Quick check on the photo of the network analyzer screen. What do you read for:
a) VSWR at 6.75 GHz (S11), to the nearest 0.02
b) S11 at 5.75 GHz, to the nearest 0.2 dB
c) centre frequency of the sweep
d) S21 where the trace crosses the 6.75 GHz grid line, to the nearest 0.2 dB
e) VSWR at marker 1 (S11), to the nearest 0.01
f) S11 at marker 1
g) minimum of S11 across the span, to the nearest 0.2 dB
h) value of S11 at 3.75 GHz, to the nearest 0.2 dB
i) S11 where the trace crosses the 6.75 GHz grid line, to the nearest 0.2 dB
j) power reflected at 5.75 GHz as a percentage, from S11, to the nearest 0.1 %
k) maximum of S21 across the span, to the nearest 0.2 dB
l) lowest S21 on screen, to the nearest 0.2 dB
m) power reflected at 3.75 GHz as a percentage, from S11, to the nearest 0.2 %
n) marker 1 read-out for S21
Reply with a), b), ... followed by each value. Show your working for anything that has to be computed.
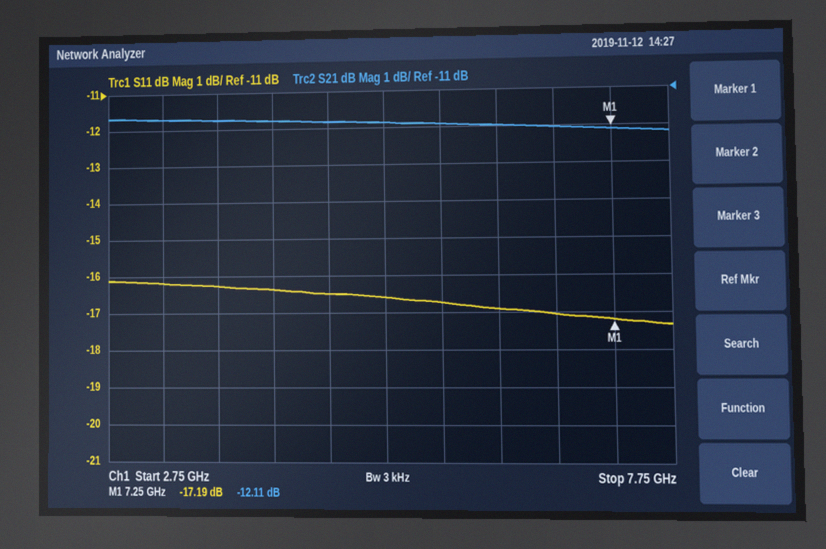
a) |Γ| = 10^(-17/20) = 0.1413; VSWR = (1 + 0.1413)/(1 − 0.1413) ≈ 1.33, so 1.32 to the nearest 0.02
b) -16.8 dB
c) 5.25 GHz
d) -12.0 dB
e) (1 + 0.1382)/(1 − 0.1382) ≈ 1.32
f) -17.19 dB
g) -17.4 dB
h) -16.2 dB
i) -17.0 dB
j) 10^(-16.8/10) ≈ 2.1 %
k) -11.6 dB
l) -12.2 dB
m) 10^(-16.2/10) ≈ 2.4 %
n) -12.11 dB
